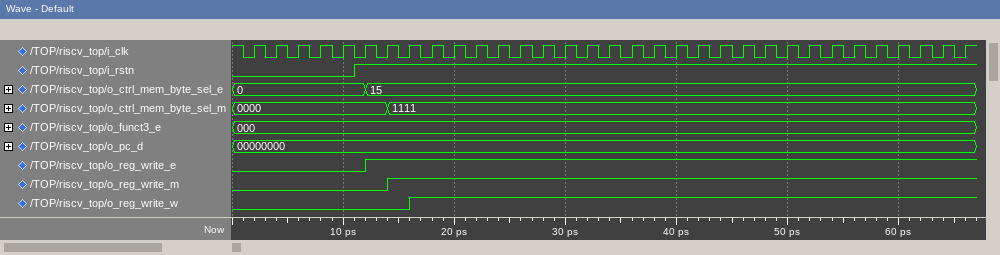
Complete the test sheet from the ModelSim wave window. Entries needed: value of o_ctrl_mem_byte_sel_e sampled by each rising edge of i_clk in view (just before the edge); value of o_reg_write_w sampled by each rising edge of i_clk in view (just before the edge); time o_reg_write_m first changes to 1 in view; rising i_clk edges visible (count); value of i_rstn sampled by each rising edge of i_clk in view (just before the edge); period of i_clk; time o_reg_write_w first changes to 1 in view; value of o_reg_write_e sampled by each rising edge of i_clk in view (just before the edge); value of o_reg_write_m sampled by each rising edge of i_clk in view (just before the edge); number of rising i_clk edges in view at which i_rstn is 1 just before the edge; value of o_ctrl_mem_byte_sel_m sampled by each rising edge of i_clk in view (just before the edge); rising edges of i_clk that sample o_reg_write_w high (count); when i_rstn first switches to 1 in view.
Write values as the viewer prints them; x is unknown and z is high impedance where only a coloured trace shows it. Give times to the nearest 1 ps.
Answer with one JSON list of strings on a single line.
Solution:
["0, 0, 0, 0, 0, 0, 15, 15, 15, 15, 15, 15, 15, 15, 15, 15, 15, 15, 15, 15, 15, 15, 15, 15, 15, 15, 15, 15, 15, 15, 15, 15, 15", "0 0 0 0 0 0 0 0 1 1 1 1 1 1 1 1 1 1 1 1 1 1 1 1 1 1 1 1 1 1 1 1 1", "14 ps", "33", "0 0 0 0 0 1 1 1 1 1 1 1 1 1 1 1 1 1 1 1 1 1 1 1 1 1 1 1 1 1 1 1 1", "2 ps", "16 ps", "0 0 0 0 0 0 1 1 1 1 1 1 1 1 1 1 1 1 1 1 1 1 1 1 1 1 1 1 1 1 1 1 1", "0 0 0 0 0 0 0 1 1 1 1 1 1 1 1 1 1 1 1 1 1 1 1 1 1 1 1 1 1 1 1 1 1", "28", "0000, 0000, 0000, 0000, 0000, 0000, 0000, 1111, 1111, 1111, 1111, 1111, 1111, 1111, 1111, 1111, 1111, 1111, 1111, 1111, 1111, 1111, 1111, 1111, 1111, 1111, 1111, 1111, 1111, 1111, 1111, 1111, 1111", "25", "11 ps"]
